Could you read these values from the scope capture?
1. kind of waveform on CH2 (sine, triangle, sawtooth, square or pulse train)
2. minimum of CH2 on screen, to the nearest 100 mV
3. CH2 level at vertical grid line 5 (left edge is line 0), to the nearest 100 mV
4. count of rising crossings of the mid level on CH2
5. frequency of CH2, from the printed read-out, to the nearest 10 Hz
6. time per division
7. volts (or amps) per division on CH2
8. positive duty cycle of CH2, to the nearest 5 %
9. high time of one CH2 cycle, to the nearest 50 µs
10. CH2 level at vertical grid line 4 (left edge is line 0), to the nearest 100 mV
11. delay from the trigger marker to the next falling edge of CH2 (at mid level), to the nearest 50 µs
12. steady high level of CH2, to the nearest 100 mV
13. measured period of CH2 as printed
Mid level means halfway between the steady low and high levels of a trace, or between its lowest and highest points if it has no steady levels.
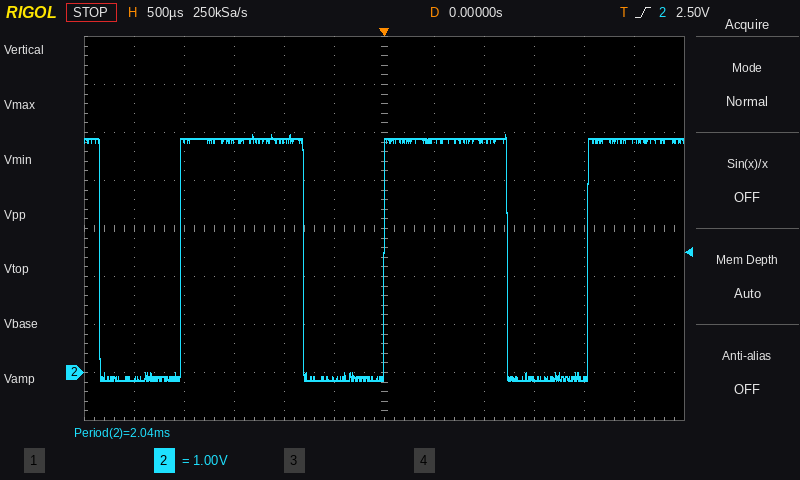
pulse train
-200 mV
-100 mV
3
490 Hz
500 µs
1 V
60 %
1.25 ms
4.8 V
1.25 ms
4.9 V
2.04 ms
